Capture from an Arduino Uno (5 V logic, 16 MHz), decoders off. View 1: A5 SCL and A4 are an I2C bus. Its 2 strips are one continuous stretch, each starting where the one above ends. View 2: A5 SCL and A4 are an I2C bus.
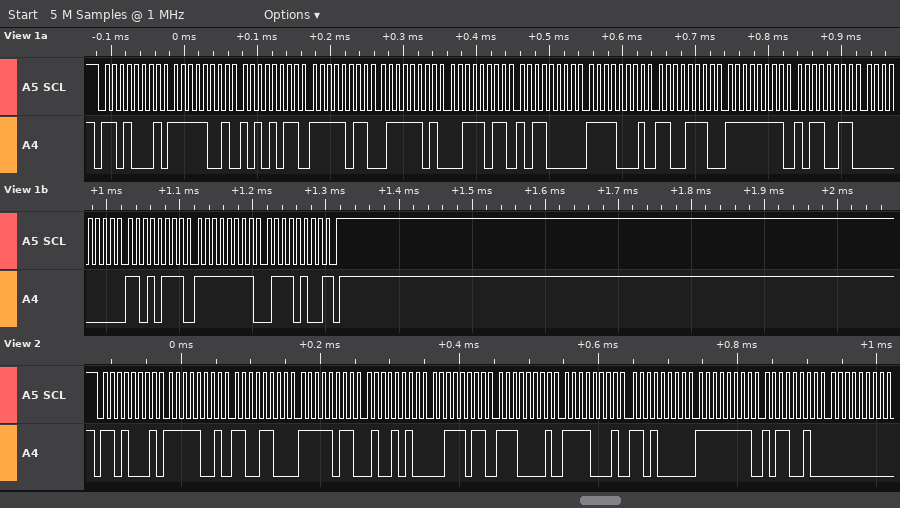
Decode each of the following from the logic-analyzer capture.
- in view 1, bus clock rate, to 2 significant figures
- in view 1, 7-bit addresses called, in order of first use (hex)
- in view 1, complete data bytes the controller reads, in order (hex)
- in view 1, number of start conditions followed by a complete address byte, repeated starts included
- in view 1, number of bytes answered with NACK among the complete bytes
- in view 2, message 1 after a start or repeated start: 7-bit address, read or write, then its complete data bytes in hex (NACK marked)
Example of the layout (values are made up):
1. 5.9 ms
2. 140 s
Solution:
1. 100 kHz
2. 0x68
3. F9 AB FB 7D 3B B0 F1 CE FF B3 00 D7 FF 74
4. 1
5. 1
6. 0x68 read: F9 CC FB 4A 3B E1 F1 D0 FF B2 00
